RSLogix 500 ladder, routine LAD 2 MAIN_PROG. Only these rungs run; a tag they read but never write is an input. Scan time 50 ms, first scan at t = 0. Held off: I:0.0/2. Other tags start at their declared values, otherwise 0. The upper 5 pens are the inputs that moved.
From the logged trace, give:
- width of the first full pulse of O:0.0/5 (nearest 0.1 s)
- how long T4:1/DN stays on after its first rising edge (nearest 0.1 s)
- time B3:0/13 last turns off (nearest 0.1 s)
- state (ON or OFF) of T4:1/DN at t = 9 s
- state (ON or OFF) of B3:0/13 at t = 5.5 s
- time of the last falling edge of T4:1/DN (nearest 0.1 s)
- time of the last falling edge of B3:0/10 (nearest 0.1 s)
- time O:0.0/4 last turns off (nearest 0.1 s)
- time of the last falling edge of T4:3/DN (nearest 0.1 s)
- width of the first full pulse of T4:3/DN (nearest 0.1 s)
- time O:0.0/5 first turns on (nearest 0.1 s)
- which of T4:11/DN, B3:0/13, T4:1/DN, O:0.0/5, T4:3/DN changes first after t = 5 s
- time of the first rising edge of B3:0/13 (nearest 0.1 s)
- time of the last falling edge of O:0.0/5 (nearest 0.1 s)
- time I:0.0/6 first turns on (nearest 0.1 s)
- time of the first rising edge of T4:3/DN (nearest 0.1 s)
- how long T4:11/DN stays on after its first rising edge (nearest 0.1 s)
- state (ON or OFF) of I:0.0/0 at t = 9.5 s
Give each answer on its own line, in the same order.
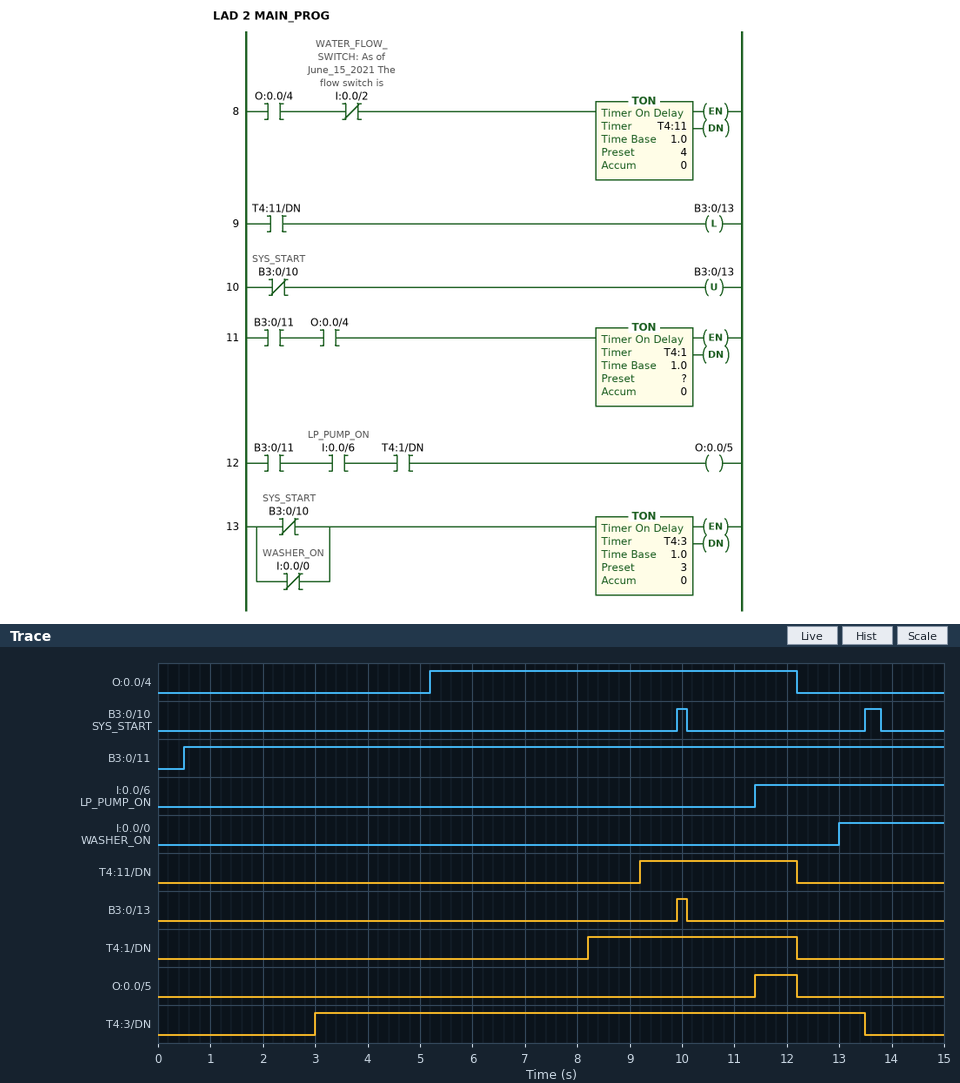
0.8 s
4.0 s
10.1 s
ON
OFF
12.2 s
13.8 s
12.2 s
13.5 s
10.5 s
11.4 s
T4:1/DN
9.9 s
12.2 s
11.4 s
3.0 s
3.0 s
OFF
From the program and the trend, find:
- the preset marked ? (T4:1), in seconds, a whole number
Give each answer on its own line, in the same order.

3 s
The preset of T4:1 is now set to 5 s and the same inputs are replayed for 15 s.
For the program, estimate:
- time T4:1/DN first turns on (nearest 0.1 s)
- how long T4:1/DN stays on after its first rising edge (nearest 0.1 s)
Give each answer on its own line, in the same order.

10.2 s
2.0 s
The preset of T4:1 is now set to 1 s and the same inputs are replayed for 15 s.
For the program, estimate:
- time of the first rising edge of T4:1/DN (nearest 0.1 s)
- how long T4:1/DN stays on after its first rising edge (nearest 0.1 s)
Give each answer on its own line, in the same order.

6.2 s
6.0 s
